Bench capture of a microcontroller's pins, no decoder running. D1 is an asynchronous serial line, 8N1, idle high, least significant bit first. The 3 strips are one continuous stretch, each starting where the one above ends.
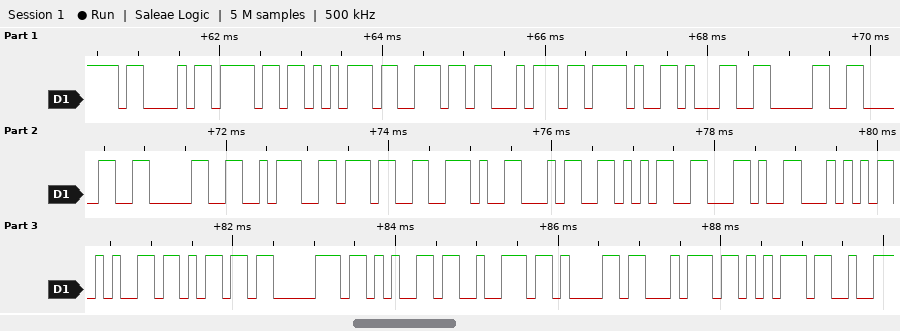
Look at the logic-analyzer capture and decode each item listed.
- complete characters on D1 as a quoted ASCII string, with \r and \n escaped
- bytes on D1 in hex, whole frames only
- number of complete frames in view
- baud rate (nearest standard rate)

"Count/1000:7.45,Temperatu"
43 6F 75 6E 74 2F 31 30 30 30 3A 37 2E 34 35 2C 54 65 6D 70 65 72 61 74 75
25
9600 baud
